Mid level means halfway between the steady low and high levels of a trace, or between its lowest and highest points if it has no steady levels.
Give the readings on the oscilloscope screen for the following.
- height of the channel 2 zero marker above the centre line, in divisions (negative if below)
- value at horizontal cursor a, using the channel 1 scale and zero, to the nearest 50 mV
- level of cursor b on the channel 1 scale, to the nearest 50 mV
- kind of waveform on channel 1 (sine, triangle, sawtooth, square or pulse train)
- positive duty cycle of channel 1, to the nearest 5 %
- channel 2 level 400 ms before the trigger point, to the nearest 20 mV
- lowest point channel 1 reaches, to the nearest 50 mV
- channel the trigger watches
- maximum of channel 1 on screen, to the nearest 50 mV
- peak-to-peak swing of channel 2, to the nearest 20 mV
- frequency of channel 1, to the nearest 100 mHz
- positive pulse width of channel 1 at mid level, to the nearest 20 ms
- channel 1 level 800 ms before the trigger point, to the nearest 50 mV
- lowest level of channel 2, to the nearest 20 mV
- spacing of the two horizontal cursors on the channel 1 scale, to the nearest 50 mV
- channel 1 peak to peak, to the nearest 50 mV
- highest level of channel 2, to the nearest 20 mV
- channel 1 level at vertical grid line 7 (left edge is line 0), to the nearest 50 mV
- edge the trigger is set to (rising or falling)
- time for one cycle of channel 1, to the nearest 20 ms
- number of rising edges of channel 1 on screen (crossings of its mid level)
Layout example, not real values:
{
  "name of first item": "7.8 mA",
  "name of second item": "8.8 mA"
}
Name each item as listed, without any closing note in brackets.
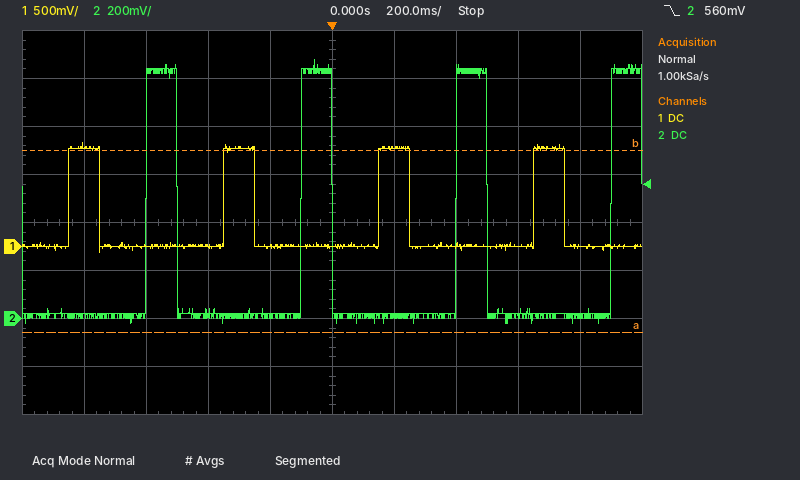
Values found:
{
  "height of the channel 2 zero marker above the centre line, in divisions": "-2.0 div",
  "value at horizontal cursor a, using the channel 1 scale and zero, to the nearest 50 mV": "-900 mV",
  "level of cursor b on the channel 1 scale, to the nearest 50 mV": "1.00 V",
  "kind of waveform on channel 1": "pulse train",
  "positive duty cycle of channel 1, to the nearest 5 %": "20 %",
  "channel 2 level 400 ms before the trigger point, to the nearest 20 mV": "20 mV",
  "lowest point channel 1 reaches, to the nearest 50 mV": "-50 mV",
  "channel the trigger watches": "channel 2",
  "maximum of channel 1 on screen, to the nearest 50 mV": "1.10 V",
  "peak-to-peak swing of channel 2, to the nearest 20 mV": "1.10 V",
  "frequency of channel 1, to the nearest 100 mHz": "2.0 Hz",
  "positive pulse width of channel 1 at mid level, to the nearest 20 ms": "100 ms",
  "channel 1 level 800 ms before the trigger point, to the nearest 50 mV": "1.05 V",
  "lowest level of channel 2, to the nearest 20 mV": "-20 mV",
  "spacing of the two horizontal cursors on the channel 1 scale, to the nearest 50 mV": "1.90 V",
  "channel 1 peak to peak, to the nearest 50 mV": "1.15 V",
  "highest level of channel 2, to the nearest 20 mV": "1.08 V",
  "channel 1 level at vertical grid line 7 (left edge is line 0), to the nearest 50 mV": "0 mV",
  "edge the trigger is set to": "falling",
  "time for one cycle of channel 1, to the nearest 20 ms": "500 ms",
  "number of rising edges of channel 1 on screen": "4"
}
